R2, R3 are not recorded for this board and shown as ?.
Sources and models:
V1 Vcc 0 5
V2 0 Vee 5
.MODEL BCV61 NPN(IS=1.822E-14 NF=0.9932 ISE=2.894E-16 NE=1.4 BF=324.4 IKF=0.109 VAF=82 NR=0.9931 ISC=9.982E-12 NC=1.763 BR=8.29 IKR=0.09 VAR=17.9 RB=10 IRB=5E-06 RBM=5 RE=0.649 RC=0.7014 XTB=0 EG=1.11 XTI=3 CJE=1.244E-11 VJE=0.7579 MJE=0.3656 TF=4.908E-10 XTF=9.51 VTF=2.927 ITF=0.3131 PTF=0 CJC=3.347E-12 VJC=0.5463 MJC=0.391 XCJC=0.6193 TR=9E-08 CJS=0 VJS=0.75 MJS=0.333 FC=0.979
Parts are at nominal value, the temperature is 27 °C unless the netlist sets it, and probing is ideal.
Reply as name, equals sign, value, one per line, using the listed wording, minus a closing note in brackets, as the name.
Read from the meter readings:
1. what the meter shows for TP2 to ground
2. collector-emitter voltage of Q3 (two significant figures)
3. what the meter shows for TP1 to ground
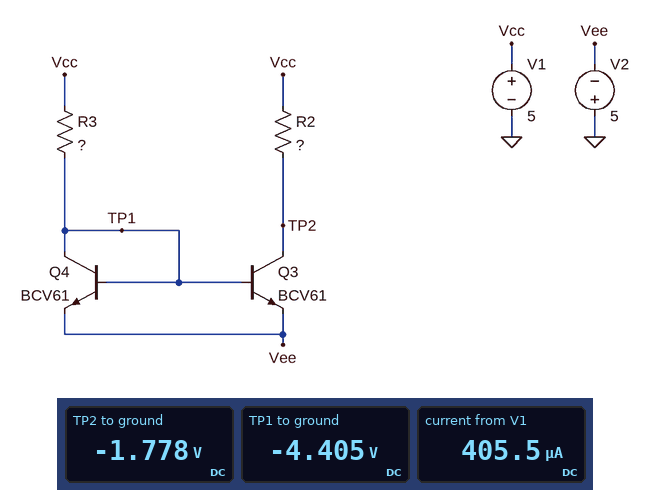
what the meter shows for TP2 to ground = -1.778 V
collector-emitter voltage of Q3 = 3.2 V
what the meter shows for TP1 to ground = -4.405 V
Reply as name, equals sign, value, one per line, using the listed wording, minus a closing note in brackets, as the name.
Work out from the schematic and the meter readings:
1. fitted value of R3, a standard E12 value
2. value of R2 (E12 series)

fitted value of R3, a standard E12 value = 47 kΩ
value of R2 = 33 kΩ
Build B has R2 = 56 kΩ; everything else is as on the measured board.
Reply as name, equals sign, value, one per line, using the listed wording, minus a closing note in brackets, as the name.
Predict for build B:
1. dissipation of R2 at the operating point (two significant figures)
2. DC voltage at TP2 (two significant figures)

dissipation of R2 at the operating point = 1.8 mW
DC voltage at TP2 = -4.9 V
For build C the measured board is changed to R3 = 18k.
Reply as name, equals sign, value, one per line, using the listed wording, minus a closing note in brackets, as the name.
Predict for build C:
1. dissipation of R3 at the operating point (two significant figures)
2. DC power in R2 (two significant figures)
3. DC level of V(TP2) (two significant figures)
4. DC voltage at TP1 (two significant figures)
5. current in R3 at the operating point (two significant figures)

dissipation of R3 at the operating point = 4.9 mW
DC power in R2 = 3.0 mW
DC level of V(TP2) = -5.0 V
DC voltage at TP1 = -4.4 V
current in R3 at the operating point = 520 µA
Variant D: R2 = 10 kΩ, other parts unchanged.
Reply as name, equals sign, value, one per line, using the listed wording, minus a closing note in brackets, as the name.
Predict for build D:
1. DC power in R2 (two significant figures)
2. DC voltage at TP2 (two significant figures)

DC power in R2 = 470 µW
DC voltage at TP2 = 2.8 V
